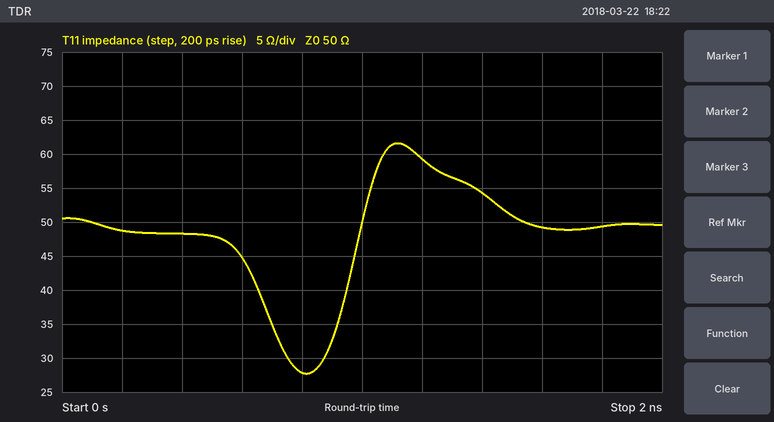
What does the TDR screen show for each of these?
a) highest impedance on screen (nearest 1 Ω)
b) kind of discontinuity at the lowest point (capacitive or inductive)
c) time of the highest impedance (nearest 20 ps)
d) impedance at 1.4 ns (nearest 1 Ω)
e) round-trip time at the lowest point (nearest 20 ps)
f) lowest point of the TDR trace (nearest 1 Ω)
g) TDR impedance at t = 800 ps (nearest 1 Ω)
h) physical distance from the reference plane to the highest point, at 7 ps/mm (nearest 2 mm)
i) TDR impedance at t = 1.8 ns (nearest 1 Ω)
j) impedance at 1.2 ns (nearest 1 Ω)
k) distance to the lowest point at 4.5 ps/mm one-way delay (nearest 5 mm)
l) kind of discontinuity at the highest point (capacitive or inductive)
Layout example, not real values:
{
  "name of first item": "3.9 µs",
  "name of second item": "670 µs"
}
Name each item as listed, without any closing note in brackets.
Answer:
{
  "highest impedance on screen": "62 Ω",
  "kind of discontinuity at the lowest point": "capacitive",
  "time of the highest impedance": "1.12 ns",
  "impedance at 1.4 ns": "54 Ω",
  "round-trip time at the lowest point": "820 ps",
  "lowest point of the TDR trace": "28 Ω",
  "TDR impedance at t = 800 ps": "28 Ω",
  "physical distance from the reference plane to the highest point, at 7 ps/mm": "80 mm",
  "TDR impedance at t = 1.8 ns": "49 Ω",
  "impedance at 1.2 ns": "59 Ω",
  "distance to the lowest point at 4.5 ps/mm one-way delay": "90 mm",
  "kind of discontinuity at the highest point": "inductive"
}
